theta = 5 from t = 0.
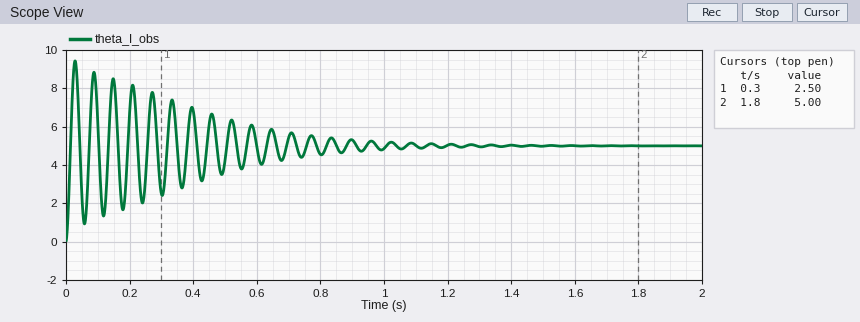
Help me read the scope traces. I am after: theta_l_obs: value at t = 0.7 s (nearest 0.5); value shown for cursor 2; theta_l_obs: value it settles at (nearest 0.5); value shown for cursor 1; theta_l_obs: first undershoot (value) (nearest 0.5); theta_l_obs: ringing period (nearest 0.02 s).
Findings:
5.5
5.00
5.0
2.50
1.0
0.06 s
